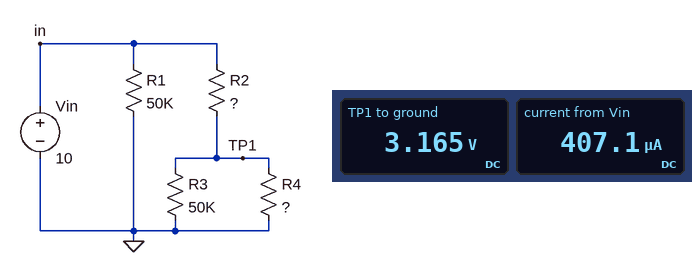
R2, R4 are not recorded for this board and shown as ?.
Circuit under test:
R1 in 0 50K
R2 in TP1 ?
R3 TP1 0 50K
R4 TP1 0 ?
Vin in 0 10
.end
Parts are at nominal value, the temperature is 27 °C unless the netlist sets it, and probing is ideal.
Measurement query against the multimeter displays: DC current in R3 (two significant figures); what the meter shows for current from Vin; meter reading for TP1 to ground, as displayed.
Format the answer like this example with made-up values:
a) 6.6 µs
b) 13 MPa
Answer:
a) 63 µA
b) 407.1 µA
c) 3.165 V
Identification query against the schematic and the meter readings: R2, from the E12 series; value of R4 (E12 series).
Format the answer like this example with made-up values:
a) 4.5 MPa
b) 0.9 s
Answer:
a) 33 kΩ
b) 22 kΩ
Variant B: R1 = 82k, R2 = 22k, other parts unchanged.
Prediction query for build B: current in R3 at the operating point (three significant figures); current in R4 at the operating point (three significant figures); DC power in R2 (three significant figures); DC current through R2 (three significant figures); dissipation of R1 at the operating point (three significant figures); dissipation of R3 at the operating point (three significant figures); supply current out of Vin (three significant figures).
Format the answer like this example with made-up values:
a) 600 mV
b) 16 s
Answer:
a) 82.0 µA
b) 186 µA
c) 1.58 mW
d) 268 µA
e) 1.22 mW
f) 336 µW
g) 390 µA
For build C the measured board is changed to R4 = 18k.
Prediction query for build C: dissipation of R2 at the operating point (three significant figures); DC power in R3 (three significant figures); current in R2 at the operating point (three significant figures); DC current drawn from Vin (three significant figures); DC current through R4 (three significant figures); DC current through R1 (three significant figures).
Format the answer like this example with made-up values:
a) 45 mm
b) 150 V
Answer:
a) 1.54 mW
b) 164 µW
c) 216 µA
d) 416 µA
e) 159 µA
f) 200 µA
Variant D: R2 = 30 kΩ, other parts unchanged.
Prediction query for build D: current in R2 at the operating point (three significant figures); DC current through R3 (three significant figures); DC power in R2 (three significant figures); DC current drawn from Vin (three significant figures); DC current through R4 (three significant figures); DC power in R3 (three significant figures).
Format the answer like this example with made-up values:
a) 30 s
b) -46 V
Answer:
a) 221 µA
b) 67.5 µA
c) 1.46 mW
d) 421 µA
e) 153 µA
f) 228 µW
